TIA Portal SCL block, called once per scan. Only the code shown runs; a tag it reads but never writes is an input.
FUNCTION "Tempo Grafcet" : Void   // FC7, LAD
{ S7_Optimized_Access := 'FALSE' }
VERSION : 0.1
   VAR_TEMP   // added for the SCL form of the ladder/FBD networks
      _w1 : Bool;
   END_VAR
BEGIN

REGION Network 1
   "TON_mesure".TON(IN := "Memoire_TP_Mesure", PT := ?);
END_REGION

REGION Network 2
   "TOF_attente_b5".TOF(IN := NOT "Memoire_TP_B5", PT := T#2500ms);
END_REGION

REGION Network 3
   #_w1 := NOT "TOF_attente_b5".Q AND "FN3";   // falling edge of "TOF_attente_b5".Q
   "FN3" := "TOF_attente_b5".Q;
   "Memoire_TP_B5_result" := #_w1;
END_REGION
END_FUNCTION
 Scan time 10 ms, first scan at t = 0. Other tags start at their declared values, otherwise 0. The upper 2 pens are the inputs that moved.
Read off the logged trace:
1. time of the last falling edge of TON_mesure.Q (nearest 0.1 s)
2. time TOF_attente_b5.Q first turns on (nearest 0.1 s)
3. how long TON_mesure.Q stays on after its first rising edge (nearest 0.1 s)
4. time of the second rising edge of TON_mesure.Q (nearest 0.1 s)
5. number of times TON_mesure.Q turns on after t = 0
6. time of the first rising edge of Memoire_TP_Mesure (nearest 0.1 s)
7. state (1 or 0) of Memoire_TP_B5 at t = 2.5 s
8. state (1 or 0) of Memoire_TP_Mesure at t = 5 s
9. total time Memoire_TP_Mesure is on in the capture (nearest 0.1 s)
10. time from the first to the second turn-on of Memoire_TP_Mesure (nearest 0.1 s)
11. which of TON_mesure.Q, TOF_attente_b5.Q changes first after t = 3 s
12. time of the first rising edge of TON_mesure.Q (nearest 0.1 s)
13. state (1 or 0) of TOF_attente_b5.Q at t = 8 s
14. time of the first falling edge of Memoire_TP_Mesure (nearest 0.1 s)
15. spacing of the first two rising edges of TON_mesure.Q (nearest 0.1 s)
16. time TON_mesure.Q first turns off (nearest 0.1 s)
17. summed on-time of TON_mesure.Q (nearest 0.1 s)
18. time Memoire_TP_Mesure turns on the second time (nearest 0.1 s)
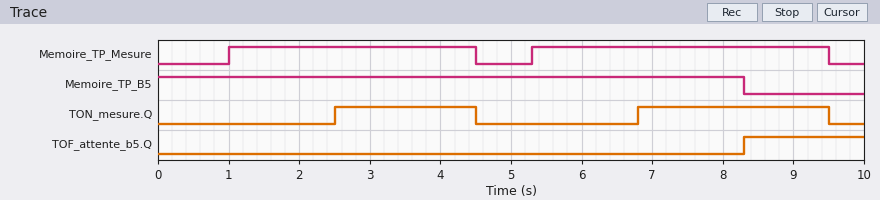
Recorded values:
9.5 s
8.3 s
2.0 s
6.8 s
2
1.0 s
1
0
7.7 s
4.3 s
TON_mesure.Q
2.5 s
0
4.5 s
4.3 s
4.5 s
4.7 s
5.3 s
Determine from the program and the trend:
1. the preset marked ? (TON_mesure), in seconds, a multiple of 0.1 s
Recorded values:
1.5 s
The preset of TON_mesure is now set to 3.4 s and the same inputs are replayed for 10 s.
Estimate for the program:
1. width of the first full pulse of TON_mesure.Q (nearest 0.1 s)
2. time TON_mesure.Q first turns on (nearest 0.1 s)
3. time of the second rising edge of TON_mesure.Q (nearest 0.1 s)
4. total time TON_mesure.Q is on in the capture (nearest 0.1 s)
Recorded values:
0.1 s
4.4 s
8.7 s
0.9 s
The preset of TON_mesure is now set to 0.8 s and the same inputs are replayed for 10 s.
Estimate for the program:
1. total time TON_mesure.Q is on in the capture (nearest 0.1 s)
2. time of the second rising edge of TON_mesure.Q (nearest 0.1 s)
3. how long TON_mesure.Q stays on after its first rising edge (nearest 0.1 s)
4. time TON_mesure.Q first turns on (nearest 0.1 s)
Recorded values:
6.1 s
6.1 s
2.7 s
1.8 s
